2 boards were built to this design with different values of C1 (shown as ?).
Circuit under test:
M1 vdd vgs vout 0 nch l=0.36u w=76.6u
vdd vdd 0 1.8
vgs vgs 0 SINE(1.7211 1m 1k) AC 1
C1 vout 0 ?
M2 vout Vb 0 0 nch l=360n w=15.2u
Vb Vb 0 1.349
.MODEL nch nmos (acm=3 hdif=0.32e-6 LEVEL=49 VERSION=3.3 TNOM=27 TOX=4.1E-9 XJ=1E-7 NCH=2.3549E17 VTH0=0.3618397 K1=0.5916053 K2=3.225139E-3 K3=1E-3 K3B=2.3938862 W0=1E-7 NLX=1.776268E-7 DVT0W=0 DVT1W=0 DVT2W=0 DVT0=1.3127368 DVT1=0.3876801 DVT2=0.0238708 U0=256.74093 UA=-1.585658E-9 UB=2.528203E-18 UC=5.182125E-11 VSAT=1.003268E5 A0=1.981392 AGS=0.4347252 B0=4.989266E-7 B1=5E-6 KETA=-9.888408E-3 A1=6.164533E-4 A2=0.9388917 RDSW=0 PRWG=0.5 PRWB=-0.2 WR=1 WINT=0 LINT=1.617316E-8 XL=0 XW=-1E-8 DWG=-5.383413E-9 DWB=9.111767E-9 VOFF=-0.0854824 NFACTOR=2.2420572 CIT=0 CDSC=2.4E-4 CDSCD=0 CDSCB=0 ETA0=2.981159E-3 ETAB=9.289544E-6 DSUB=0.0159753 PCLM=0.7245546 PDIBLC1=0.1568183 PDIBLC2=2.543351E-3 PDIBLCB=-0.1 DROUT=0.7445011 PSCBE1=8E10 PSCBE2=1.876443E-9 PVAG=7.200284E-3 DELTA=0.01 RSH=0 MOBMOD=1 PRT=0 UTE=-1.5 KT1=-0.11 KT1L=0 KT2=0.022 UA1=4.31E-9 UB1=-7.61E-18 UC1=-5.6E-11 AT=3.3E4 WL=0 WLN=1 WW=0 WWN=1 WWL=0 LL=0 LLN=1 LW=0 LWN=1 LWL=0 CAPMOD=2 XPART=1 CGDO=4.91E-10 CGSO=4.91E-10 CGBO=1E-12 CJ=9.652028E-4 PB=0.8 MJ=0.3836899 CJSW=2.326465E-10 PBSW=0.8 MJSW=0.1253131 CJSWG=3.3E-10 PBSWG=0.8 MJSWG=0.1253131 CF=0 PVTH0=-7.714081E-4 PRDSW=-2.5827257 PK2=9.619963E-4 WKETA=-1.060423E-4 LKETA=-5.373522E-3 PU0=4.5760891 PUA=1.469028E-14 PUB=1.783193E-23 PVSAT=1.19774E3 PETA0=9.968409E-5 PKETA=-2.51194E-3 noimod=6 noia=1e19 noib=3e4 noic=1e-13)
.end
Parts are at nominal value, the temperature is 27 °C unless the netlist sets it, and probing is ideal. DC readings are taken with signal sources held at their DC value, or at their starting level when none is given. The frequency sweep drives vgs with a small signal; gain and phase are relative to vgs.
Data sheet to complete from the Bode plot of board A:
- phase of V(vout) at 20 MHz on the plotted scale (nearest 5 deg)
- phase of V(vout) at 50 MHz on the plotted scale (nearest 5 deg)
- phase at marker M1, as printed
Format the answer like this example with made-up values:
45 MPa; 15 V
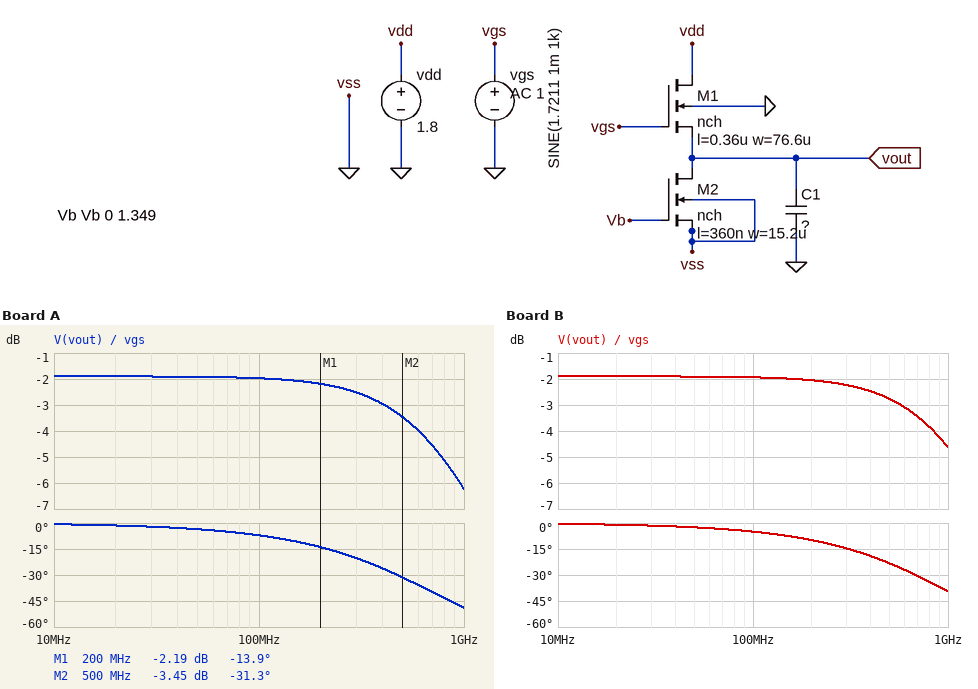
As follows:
0 deg; -5 deg; -13.9 deg
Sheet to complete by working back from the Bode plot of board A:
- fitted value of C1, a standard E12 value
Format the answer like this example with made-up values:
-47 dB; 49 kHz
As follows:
3.9 pF
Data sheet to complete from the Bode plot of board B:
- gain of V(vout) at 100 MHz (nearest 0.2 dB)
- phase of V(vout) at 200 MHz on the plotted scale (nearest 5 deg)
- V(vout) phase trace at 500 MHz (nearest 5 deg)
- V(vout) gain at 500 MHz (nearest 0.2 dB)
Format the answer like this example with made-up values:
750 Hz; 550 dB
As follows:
-2.0 dB; -10 deg; -25 deg; -2.8 dB
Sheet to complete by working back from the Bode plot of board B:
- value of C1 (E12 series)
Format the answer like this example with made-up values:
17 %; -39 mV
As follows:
2.7 pF
